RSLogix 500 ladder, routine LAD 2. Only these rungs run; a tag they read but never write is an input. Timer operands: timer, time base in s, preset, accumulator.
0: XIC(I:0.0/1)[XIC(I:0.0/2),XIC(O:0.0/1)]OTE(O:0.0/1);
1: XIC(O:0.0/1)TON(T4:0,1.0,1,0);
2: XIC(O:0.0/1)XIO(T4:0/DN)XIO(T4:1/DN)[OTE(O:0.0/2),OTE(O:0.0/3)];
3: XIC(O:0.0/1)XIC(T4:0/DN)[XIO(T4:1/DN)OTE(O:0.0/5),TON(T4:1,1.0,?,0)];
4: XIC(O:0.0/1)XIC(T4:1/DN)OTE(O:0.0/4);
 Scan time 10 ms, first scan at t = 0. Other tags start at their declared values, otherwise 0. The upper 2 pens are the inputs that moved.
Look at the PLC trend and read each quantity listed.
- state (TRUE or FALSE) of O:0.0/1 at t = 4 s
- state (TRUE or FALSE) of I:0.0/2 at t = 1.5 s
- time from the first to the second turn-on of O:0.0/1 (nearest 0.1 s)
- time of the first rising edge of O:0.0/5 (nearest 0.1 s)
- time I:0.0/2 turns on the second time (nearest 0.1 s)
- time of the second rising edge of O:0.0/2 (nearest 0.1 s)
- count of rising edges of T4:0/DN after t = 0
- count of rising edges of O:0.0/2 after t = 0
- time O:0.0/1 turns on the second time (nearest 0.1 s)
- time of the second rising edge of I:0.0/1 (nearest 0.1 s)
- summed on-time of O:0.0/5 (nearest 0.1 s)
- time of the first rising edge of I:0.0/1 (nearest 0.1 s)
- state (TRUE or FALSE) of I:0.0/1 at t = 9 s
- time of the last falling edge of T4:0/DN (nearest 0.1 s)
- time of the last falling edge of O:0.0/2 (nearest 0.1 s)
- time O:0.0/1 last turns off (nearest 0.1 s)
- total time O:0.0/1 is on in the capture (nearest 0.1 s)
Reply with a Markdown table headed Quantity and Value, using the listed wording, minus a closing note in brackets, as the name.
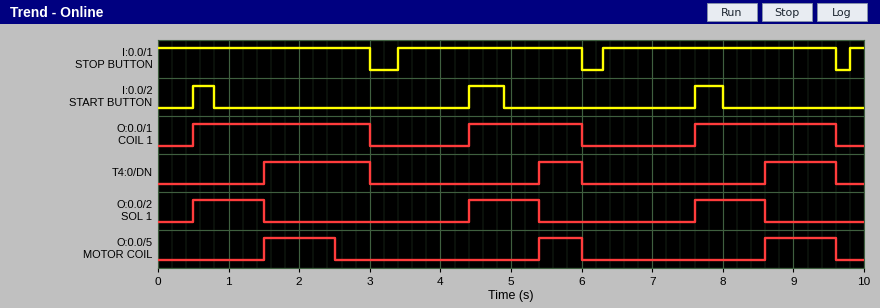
| Quantity | Value |
|---|---|
| state (TRUE or FALSE) of O:0.0/1 at t = 4 s | FALSE |
| state (TRUE or FALSE) of I:0.0/2 at t = 1.5 s | FALSE |
| time from the first to the second turn-on of O:0.0/1 | 3.9 s |
| time of the first rising edge of O:0.0/5 | 1.5 s |
| time I:0.0/2 turns on the second time | 4.4 s |
| time of the second rising edge of O:0.0/2 | 4.4 s |
| count of rising edges of T4:0/DN after t = 0 | 3 |
| count of rising edges of O:0.0/2 after t = 0 | 3 |
| time O:0.0/1 turns on the second time | 4.4 s |
| time of the second rising edge of I:0.0/1 | 6.3 s |
| summed on-time of O:0.0/5 | 2.6 s |
| time of the first rising edge of I:0.0/1 | 3.4 s |
| state (TRUE or FALSE) of I:0.0/1 at t = 9 s | TRUE |
| time of the last falling edge of T4:0/DN | 9.6 s |
| time of the last falling edge of O:0.0/2 | 8.6 s |
| time O:0.0/1 last turns off | 9.6 s |
| total time O:0.0/1 is on in the capture | 6.1 s |
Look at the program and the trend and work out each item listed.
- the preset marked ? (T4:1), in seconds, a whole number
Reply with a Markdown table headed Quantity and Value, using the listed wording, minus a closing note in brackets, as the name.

| Quantity | Value |
|---|---|
| the preset marked ? (T4:1), in seconds, a whole number | 1 s |
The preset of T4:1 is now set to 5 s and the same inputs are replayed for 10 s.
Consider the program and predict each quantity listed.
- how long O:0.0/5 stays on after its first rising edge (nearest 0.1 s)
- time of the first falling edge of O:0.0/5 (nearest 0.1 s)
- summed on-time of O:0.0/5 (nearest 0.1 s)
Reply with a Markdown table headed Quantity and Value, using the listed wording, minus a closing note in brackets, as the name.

| Quantity | Value |
|---|---|
| how long O:0.0/5 stays on after its first rising edge | 1.5 s |
| time of the first falling edge of O:0.0/5 | 3.0 s |
| summed on-time of O:0.0/5 | 3.1 s |
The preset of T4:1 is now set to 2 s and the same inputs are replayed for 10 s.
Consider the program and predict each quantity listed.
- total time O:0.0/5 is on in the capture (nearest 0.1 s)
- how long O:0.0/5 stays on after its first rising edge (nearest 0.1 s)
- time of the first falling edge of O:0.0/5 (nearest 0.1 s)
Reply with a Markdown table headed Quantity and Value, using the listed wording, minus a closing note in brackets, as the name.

| Quantity | Value |
|---|---|
| total time O:0.0/5 is on in the capture | 3.1 s |
| how long O:0.0/5 stays on after its first rising edge | 1.5 s |
| time of the first falling edge of O:0.0/5 | 3.0 s |
